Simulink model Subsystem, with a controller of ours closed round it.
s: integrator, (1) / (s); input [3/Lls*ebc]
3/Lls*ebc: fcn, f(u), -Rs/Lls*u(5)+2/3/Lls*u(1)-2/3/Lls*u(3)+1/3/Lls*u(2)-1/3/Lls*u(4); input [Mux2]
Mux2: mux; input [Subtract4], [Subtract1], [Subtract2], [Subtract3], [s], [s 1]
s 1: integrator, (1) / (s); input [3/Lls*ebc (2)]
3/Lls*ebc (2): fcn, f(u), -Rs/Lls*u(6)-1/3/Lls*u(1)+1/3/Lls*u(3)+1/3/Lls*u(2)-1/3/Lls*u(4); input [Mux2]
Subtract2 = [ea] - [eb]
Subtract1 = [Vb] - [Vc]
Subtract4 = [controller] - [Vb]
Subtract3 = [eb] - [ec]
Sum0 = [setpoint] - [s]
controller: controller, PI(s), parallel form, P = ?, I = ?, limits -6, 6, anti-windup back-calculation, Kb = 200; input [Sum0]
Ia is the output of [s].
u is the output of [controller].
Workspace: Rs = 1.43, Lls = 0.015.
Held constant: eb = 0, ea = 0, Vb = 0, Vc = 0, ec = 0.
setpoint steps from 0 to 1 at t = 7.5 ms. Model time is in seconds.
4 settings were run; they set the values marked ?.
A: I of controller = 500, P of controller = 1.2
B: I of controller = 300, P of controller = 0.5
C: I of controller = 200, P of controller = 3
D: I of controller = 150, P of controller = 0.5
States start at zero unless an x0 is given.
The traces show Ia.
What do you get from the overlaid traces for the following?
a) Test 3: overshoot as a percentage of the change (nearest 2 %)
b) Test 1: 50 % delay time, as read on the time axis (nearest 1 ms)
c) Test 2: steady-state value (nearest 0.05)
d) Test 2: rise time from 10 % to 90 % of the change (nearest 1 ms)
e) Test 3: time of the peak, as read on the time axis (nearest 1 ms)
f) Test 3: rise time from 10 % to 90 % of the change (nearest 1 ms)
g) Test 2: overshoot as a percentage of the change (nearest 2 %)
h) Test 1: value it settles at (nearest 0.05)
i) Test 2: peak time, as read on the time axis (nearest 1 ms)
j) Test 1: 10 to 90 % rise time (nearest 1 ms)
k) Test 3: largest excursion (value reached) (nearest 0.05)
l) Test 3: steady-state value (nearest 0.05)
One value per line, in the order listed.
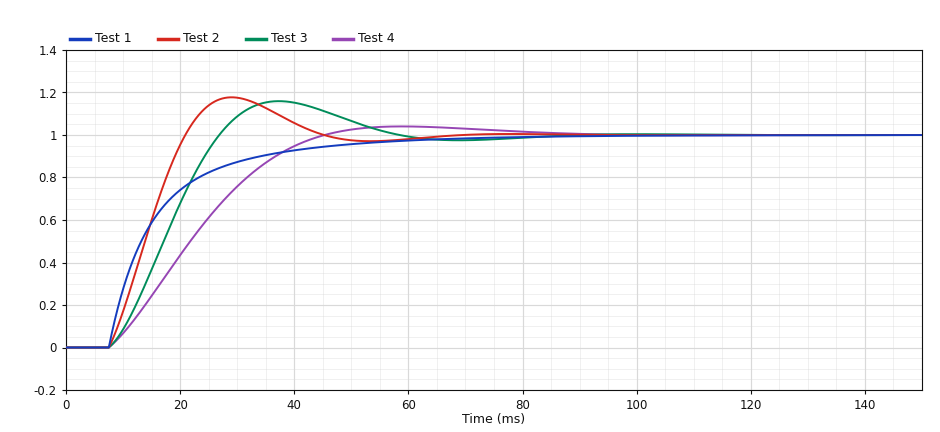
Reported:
16 %
13 ms
1.00
10 ms
37 ms
14 ms
18 %
1.00
29 ms
26 ms
1.15
1.00
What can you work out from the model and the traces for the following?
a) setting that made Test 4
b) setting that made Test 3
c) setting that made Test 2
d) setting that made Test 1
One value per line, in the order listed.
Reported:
D
B
A
C
